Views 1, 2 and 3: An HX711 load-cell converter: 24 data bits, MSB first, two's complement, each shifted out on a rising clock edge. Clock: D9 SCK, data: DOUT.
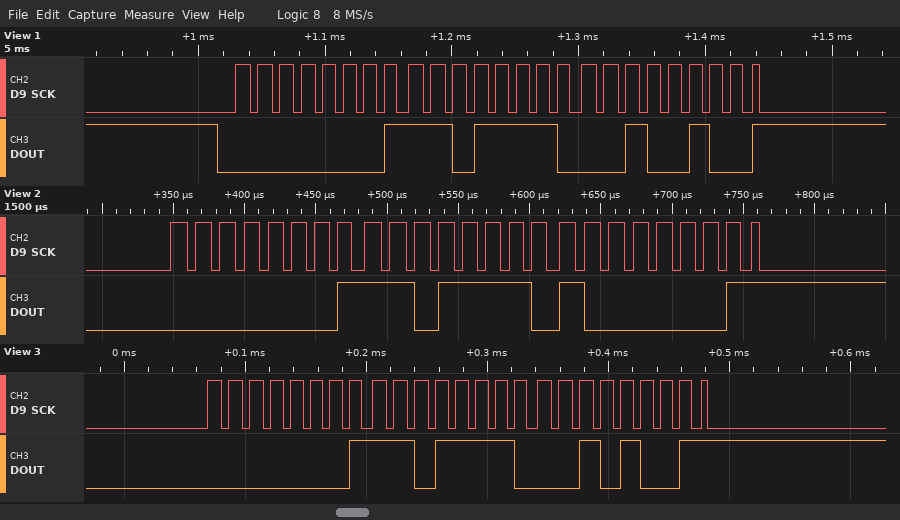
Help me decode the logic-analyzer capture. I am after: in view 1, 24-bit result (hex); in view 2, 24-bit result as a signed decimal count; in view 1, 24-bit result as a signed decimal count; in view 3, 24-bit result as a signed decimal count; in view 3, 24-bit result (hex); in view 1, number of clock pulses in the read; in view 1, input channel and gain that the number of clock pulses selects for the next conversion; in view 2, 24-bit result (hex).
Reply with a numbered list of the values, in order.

1. 0x01DE24
2. 122497
3. 122404
4. 122409
5. 0x01DE29
6. 25
7. channel A, gain 128
8. 0x01DE81
